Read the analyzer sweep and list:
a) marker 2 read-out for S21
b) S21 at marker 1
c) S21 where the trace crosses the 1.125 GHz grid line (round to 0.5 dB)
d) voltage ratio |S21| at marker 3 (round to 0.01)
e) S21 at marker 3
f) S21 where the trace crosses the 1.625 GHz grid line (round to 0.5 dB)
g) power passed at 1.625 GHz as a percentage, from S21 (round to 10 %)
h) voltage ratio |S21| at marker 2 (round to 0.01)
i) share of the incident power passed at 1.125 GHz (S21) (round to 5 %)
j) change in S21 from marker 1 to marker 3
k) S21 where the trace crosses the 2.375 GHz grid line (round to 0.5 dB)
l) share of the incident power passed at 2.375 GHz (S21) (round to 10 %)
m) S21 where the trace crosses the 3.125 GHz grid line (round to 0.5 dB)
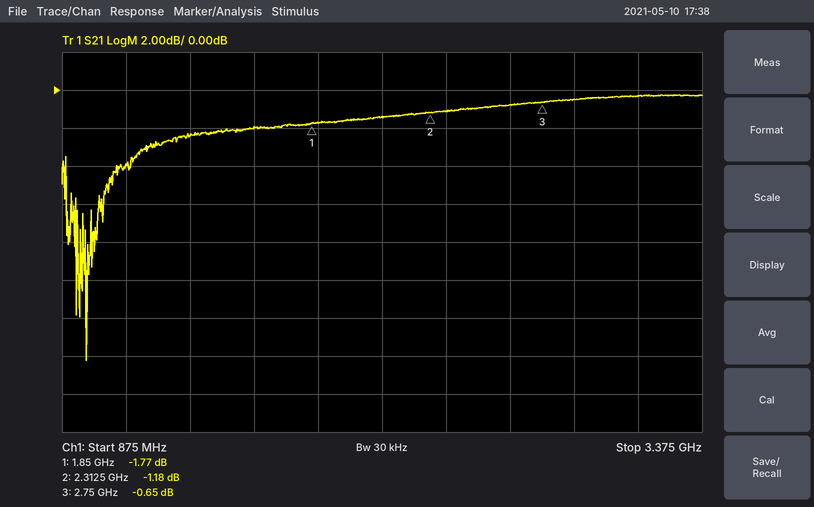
-1.18 dB
-1.77 dB
-4.0 dB
0.93
-0.65 dB
-2.0 dB
60 %
0.87
40 %
1.12 dB
-1.0 dB
80 %
-0.5 dB
